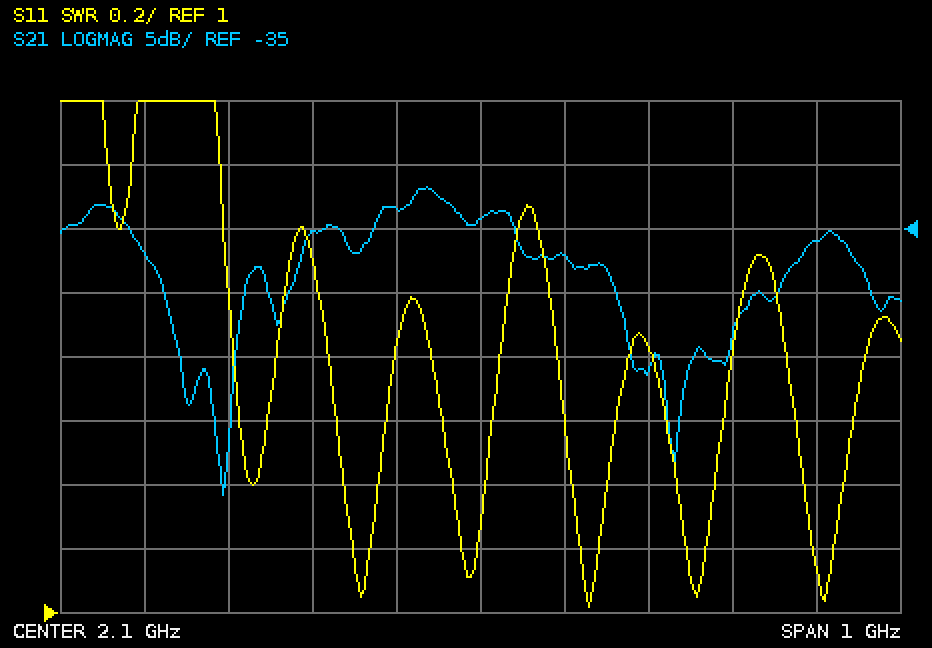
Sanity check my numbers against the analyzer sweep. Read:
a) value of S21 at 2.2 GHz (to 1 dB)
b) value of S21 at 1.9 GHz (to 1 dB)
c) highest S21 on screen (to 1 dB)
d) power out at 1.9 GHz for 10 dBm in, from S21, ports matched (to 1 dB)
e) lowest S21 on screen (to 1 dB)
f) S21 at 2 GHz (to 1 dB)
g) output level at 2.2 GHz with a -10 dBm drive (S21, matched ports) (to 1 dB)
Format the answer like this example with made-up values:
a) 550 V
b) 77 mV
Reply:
a) -37 dB
b) -35 dB
c) -32 dB
d) -25 dBm
e) -56 dB
f) -33 dB
g) -47 dBm
